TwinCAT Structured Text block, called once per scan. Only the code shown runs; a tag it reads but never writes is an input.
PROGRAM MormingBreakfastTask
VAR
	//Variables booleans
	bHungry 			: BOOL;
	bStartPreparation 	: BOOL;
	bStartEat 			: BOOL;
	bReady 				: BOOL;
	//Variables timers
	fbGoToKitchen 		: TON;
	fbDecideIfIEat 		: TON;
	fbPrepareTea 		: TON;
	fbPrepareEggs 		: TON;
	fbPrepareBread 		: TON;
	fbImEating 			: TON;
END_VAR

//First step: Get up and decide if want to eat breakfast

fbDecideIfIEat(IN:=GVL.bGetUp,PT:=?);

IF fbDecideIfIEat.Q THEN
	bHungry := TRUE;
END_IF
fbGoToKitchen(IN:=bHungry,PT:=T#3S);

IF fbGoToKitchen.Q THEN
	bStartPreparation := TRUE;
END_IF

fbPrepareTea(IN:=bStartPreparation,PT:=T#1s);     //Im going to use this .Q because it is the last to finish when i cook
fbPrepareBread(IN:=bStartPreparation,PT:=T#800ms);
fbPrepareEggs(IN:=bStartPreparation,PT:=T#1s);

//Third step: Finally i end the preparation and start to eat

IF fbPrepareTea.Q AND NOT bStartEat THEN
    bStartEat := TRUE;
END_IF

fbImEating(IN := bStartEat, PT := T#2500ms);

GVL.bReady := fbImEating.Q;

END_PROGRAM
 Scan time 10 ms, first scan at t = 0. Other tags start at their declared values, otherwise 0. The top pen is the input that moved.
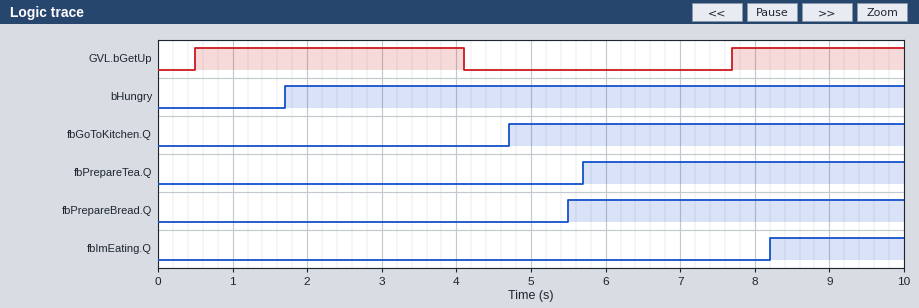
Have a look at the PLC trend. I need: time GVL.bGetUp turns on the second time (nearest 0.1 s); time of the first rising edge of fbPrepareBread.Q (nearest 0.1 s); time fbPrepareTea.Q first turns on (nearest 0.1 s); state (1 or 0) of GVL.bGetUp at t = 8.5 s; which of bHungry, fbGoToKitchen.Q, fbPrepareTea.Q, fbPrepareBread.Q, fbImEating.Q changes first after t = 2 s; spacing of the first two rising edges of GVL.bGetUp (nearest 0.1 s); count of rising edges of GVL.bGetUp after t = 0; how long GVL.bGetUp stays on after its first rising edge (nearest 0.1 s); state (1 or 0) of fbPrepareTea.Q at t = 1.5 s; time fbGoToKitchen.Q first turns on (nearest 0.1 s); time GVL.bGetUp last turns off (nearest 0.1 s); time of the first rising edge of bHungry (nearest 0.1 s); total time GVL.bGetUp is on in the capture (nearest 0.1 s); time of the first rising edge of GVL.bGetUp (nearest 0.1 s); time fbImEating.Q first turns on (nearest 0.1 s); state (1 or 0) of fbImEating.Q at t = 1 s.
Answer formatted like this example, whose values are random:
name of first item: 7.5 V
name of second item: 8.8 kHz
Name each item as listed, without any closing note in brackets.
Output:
time GVL.bGetUp turns on the second time: 7.7 s
time of the first rising edge of fbPrepareBread.Q: 5.5 s
time fbPrepareTea.Q first turns on: 5.7 s
state (1 or 0) of GVL.bGetUp at t = 8.5 s: 1
which of bHungry, fbGoToKitchen.Q, fbPrepareTea.Q, fbPrepareBread.Q, fbImEating.Q changes first after t = 2 s: fbGoToKitchen.Q
spacing of the first two rising edges of GVL.bGetUp: 7.2 s
count of rising edges of GVL.bGetUp after t = 0: 2
how long GVL.bGetUp stays on after its first rising edge: 3.6 s
state (1 or 0) of fbPrepareTea.Q at t = 1.5 s: 0
time fbGoToKitchen.Q first turns on: 4.7 s
time GVL.bGetUp last turns off: 4.1 s
time of the first rising edge of bHungry: 1.7 s
total time GVL.bGetUp is on in the capture: 5.9 s
time of the first rising edge of GVL.bGetUp: 0.5 s
time fbImEating.Q first turns on: 8.2 s
state (1 or 0) of fbImEating.Q at t = 1 s: 0
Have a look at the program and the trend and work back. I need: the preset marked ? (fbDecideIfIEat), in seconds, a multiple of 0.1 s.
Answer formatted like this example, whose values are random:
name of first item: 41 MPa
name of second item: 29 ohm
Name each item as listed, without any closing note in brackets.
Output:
the preset marked ? (fbDecideIfIEat), in seconds, a multiple of 0.1 s: 1.2 s
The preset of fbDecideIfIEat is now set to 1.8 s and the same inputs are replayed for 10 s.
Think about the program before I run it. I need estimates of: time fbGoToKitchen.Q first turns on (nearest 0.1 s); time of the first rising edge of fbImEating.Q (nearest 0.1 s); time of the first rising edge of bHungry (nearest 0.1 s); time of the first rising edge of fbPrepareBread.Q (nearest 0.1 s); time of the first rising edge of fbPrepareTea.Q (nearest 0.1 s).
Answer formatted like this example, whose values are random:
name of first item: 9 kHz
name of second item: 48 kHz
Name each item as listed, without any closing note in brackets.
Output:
time fbGoToKitchen.Q first turns on: 5.3 s
time of the first rising edge of fbImEating.Q: 8.8 s
time of the first rising edge of bHungry: 2.3 s
time of the first rising edge of fbPrepareBread.Q: 6.1 s
time of the first rising edge of fbPrepareTea.Q: 6.3 s
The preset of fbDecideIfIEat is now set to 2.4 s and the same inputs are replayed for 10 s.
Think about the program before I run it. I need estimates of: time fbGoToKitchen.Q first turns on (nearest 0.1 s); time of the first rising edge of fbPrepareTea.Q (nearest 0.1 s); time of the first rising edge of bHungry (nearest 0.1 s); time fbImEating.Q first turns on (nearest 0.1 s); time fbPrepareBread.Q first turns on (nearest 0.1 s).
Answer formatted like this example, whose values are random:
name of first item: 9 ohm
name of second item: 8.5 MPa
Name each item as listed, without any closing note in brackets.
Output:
time fbGoToKitchen.Q first turns on: 5.9 s
time of the first rising edge of fbPrepareTea.Q: 6.9 s
time of the first rising edge of bHungry: 2.9 s
time fbImEating.Q first turns on: 9.4 s
time fbPrepareBread.Q first turns on: 6.7 s
